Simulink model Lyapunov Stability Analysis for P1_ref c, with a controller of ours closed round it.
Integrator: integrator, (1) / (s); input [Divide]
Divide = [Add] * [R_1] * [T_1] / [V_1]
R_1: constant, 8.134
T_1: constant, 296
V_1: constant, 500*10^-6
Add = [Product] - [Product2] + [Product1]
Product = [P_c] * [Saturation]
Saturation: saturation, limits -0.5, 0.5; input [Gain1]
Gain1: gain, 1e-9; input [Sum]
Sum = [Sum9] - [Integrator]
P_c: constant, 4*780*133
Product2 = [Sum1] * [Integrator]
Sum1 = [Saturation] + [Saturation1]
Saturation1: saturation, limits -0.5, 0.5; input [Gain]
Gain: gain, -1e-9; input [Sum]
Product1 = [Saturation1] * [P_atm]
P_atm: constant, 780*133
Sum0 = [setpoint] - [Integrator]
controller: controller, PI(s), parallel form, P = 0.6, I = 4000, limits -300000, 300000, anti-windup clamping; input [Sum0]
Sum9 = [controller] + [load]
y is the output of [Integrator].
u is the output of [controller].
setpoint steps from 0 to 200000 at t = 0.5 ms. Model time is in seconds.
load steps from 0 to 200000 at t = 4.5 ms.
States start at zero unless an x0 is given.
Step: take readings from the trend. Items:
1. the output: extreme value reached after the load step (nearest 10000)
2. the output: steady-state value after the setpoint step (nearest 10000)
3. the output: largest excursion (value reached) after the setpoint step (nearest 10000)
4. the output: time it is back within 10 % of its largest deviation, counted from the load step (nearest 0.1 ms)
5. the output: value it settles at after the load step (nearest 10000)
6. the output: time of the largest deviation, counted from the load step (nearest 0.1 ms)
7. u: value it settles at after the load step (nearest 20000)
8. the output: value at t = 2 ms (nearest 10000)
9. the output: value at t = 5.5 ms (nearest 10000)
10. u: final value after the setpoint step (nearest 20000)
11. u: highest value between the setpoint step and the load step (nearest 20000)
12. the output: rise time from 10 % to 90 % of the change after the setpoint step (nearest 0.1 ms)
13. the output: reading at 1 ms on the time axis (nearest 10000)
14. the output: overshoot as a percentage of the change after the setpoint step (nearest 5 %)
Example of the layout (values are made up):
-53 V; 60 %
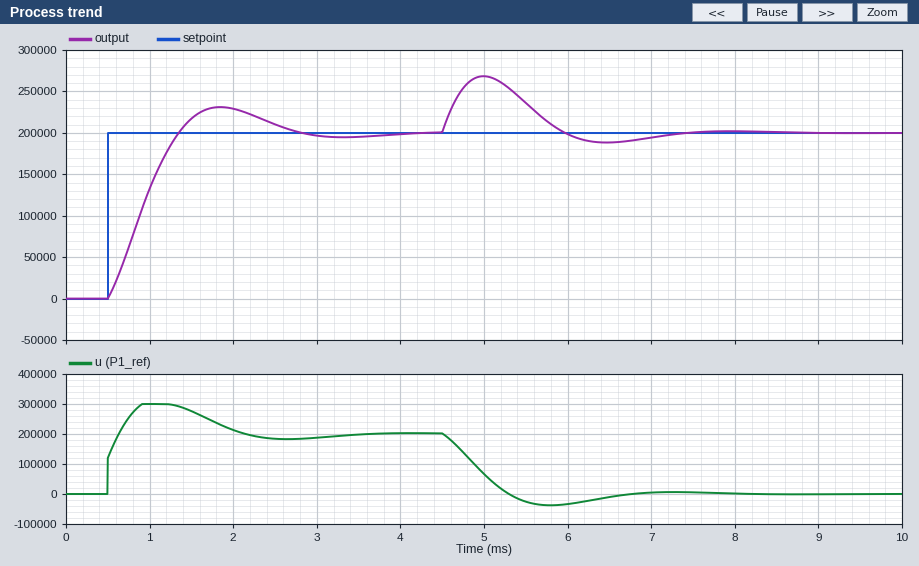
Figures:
270000; 200000; 230000; 2.4 ms; 200000; 0.5 ms; 0; 230000; 240000; 200000; 300000; 0.6 ms; 130000; 15 %
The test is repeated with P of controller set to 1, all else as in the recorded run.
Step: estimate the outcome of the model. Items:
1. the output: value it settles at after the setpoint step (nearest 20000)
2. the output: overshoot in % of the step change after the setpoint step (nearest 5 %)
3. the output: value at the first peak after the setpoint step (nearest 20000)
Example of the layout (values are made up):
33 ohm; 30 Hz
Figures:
200000; 10 %; 220000
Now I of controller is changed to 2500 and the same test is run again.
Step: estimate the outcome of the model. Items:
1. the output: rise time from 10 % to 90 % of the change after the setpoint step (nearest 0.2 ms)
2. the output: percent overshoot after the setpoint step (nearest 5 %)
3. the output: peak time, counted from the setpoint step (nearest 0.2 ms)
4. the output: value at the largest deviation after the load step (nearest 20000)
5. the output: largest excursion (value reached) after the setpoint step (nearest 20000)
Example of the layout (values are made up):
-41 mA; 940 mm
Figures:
0.8 ms; 10 %; 1.8 ms; 280000; 220000
